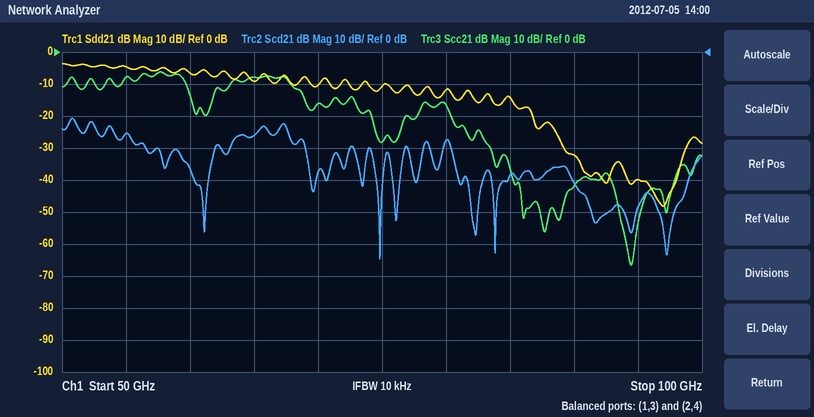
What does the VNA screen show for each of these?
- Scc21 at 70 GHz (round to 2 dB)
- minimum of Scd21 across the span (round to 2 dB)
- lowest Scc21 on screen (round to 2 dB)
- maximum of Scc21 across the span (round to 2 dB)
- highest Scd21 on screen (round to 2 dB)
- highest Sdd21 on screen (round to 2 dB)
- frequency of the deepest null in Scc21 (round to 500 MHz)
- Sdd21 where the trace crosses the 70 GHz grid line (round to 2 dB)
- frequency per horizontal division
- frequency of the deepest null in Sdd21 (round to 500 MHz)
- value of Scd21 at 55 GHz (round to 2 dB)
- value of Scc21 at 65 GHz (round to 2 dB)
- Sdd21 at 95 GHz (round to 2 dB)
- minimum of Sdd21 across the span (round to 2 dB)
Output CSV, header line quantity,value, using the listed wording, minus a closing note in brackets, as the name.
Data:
quantity,value
Scc21 at 70 GHz,-16 dB
minimum of Scd21 across the span,-64 dB
lowest Scc21 on screen,-66 dB
maximum of Scc21 across the span,-6 dB
highest Scd21 on screen,-20 dB
highest Sdd21 on screen,-4 dB
frequency of the deepest null in Scc21,94.5 GHz
Sdd21 where the trace crosses the 70 GHz grid line,-10 dB
frequency per horizontal division,5 GHz
frequency of the deepest null in Sdd21,97.0 GHz
value of Scd21 at 55 GHz,-26 dB
value of Scc21 at 65 GHz,-8 dB
Sdd21 at 95 GHz,-40 dB
minimum of Sdd21 across the span,-48 dB
